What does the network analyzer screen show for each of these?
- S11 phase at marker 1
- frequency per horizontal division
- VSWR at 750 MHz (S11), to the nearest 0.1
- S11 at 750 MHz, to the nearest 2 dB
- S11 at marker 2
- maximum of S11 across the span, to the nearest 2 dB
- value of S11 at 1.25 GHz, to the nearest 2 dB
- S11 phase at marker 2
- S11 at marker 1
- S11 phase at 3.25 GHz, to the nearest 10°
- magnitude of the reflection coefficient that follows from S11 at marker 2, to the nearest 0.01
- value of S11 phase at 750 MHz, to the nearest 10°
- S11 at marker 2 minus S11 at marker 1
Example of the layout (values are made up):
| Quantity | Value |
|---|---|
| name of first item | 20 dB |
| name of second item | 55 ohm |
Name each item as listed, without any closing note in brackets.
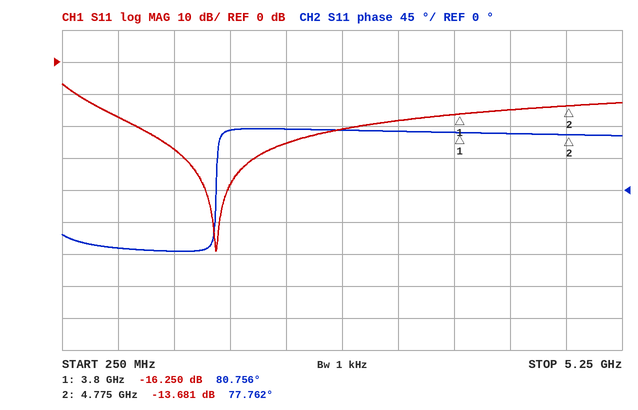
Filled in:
| Quantity | Value |
|---|---|
| S11 phase at marker 1 | 80.756° |
| frequency per horizontal division | 500 MHz |
| VSWR at 750 MHz (S11), to the nearest 0.1 | 1.3 |
| S11 at 750 MHz, to the nearest 2 dB | -18 dB |
| S11 at marker 2 | -13.681 dB |
| maximum of S11 across the span, to the nearest 2 dB | -6 dB |
| value of S11 at 1.25 GHz, to the nearest 2 dB | -28 dB |
| S11 phase at marker 2 | 77.762° |
| S11 at marker 1 | -16.250 dB |
| S11 phase at 3.25 GHz, to the nearest 10° | 80° |
| magnitude of the reflection coefficient that follows from S11 at marker 2, to the nearest 0.01 | 0.21 |
| value of S11 phase at 750 MHz, to the nearest 10° | -80° |
| S11 at marker 2 minus S11 at marker 1 | 2.569 dB |
